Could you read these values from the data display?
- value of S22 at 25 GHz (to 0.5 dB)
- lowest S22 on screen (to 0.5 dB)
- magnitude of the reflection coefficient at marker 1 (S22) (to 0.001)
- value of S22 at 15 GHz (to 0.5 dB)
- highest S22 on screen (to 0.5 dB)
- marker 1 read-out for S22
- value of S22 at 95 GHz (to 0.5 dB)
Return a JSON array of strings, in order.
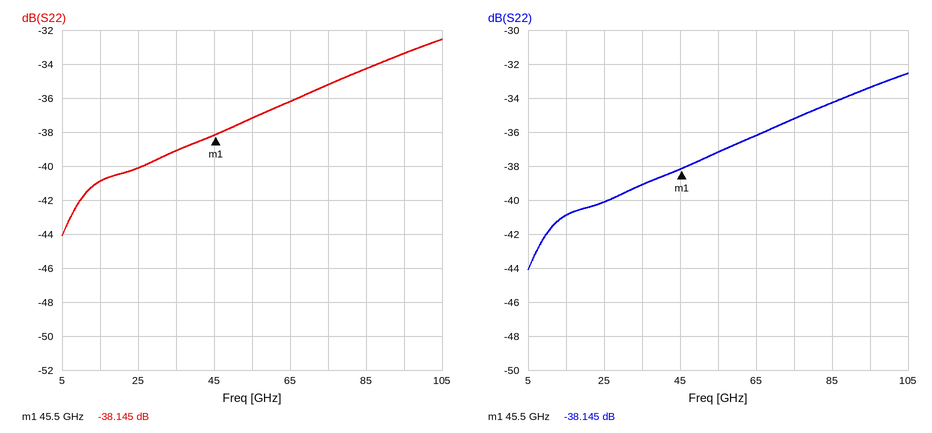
["-40.0 dB", "-44.0 dB", "0.012", "-41.0 dB", "-32.5 dB", "-38.145 dB", "-33.5 dB"]
